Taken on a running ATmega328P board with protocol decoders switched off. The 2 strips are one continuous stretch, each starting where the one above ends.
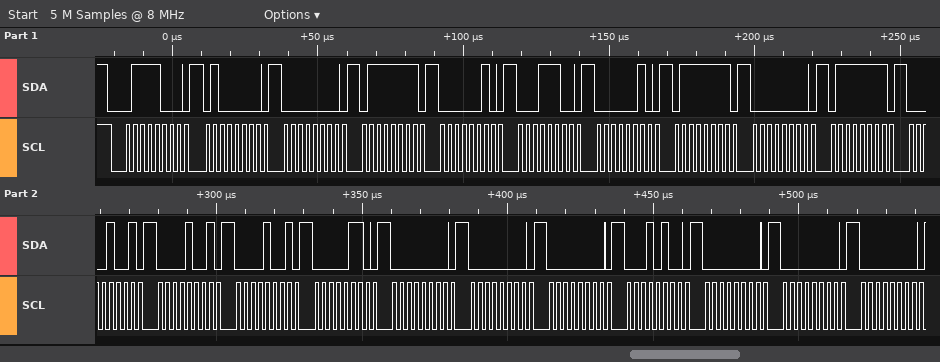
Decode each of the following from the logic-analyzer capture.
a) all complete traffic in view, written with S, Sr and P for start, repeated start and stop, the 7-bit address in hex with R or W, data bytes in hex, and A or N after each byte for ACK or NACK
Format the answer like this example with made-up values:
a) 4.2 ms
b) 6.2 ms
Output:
a) S 3CW A 40 A 00 A 7F A 02 A 1C A 02 A 7F A 00 A 7F A 09 A 09 A 09 A 06 A 00 A 00 A 00 A 14 A 00 A 00 A 00 A
